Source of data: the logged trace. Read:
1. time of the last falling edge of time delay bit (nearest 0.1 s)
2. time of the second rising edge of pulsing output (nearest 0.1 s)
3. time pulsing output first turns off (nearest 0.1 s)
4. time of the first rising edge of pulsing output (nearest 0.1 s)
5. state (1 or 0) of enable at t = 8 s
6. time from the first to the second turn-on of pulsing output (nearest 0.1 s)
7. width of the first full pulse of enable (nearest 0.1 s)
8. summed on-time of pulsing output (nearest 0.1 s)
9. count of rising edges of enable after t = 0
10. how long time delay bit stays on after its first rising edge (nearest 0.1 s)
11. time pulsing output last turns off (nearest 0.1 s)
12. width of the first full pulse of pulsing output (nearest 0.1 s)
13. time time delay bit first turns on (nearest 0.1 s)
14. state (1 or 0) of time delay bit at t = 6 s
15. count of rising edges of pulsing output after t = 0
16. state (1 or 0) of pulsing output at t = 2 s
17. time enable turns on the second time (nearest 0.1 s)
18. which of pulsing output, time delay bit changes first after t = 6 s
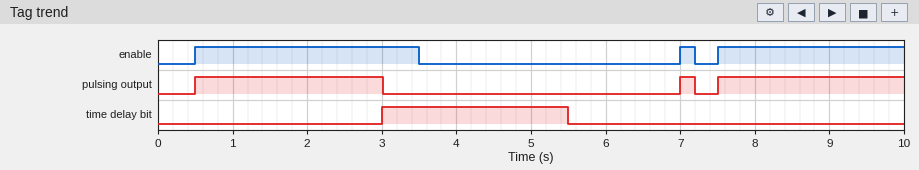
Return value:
5.5 s
7.0 s
3.0 s
0.5 s
1
6.5 s
3.0 s
5.2 s
3
2.5 s
7.2 s
2.5 s
3.0 s
0
3
1
7.0 s
pulsing output
